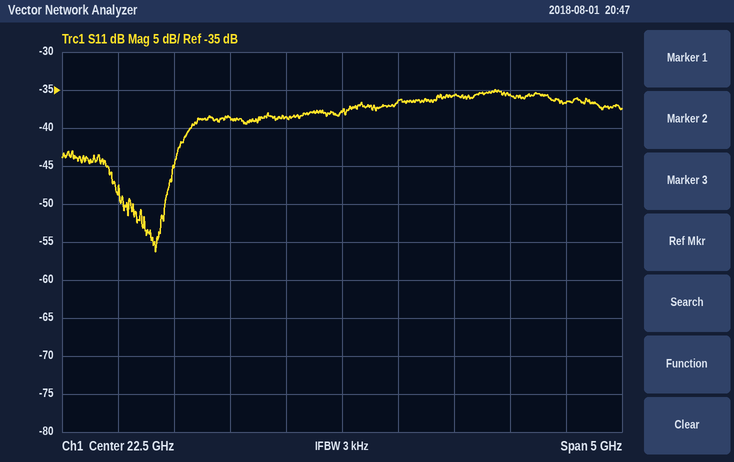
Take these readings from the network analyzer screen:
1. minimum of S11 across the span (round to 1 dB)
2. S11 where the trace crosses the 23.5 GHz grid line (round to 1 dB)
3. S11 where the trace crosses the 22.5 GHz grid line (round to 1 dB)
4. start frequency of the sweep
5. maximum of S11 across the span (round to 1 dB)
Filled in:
-56 dB
-36 dB
-38 dB
20 GHz
-35 dB
